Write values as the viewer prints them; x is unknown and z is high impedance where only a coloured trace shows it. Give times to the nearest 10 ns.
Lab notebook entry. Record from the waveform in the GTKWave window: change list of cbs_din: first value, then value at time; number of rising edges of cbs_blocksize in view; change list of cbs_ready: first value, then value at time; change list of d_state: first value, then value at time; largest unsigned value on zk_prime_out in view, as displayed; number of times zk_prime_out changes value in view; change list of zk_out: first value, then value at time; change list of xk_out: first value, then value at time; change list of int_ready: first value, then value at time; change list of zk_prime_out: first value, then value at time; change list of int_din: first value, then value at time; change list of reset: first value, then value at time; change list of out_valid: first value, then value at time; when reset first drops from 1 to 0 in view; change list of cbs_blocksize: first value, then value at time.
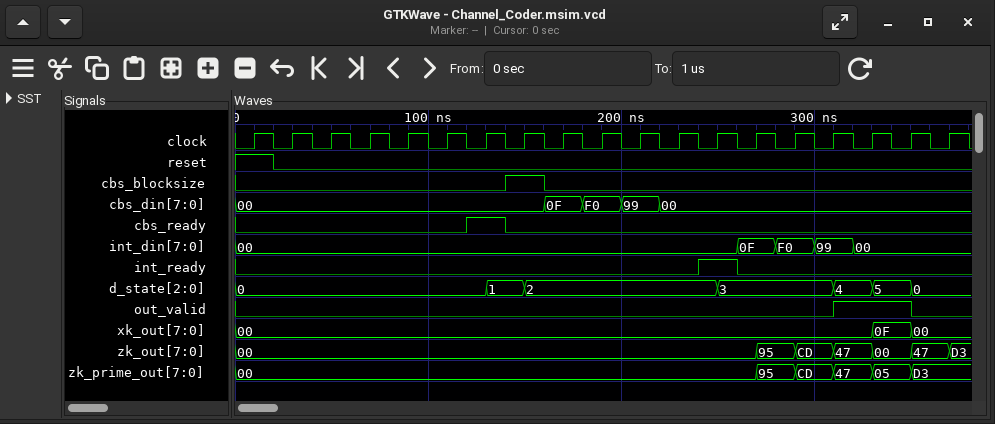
00, 0F at 160 ns, F0 at 180 ns, 99 at 200 ns, 00 at 220 ns
1
0, 1 at 120 ns, 0 at 140 ns
0, 1 at 130 ns, 2 at 150 ns, 3 at 250 ns, 4 at 310 ns, 5 at 330 ns, 0 at 350 ns
D3
5
00, 95 at 270 ns, CD at 290 ns, 47 at 310 ns, 00 at 330 ns, 47 at 350 ns, D3 at 370 ns
00, 0F at 330 ns, 00 at 350 ns
0, 1 at 240 ns, 0 at 260 ns
00, 95 at 270 ns, CD at 290 ns, 47 at 310 ns, 05 at 330 ns, D3 at 350 ns
00, 0F at 260 ns, F0 at 280 ns, 99 at 300 ns, 00 at 320 ns
1, 0 at 20 ns
0, 1 at 310 ns, 0 at 350 ns
20 ns
0, 1 at 140 ns, 0 at 160 ns
